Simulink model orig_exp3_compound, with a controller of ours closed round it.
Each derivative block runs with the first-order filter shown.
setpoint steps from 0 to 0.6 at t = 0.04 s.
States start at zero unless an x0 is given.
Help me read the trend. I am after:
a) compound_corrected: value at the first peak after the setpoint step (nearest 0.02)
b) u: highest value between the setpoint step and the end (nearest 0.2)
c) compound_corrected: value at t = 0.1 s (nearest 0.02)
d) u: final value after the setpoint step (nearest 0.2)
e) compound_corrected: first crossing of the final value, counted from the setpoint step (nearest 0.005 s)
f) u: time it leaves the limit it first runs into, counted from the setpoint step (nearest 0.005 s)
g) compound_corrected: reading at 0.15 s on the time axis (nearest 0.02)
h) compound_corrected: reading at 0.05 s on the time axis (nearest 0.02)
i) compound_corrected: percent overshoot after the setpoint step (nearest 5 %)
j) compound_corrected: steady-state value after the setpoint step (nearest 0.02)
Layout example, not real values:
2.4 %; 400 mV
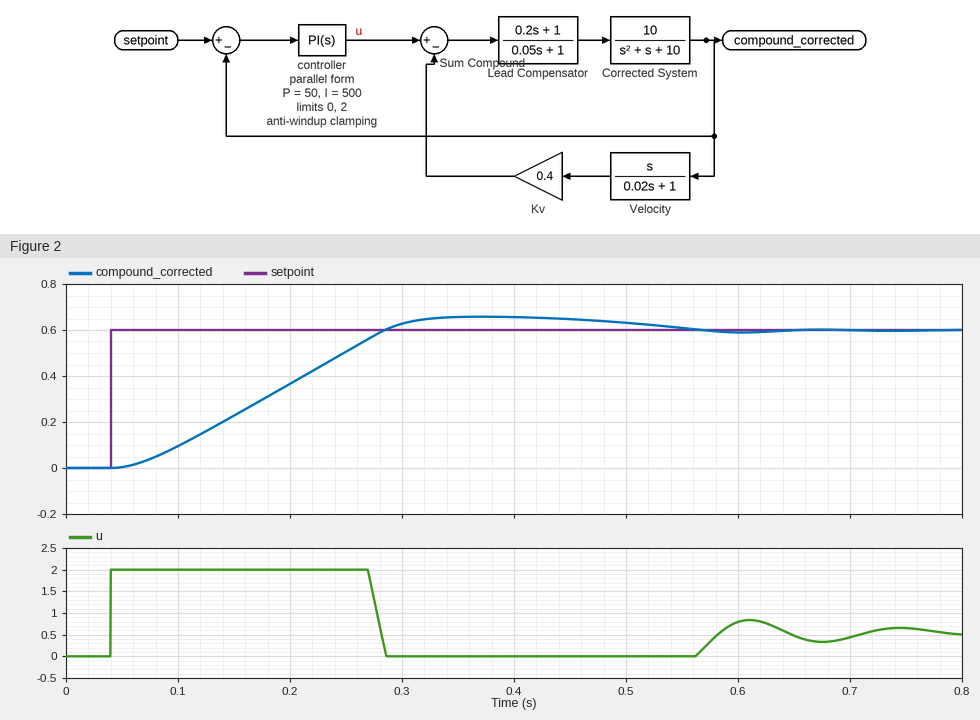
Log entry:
0.66; 2.0; 0.10; 0.6; 0.245 s; 0.230 s; 0.22; 0.00; 10 %; 0.60
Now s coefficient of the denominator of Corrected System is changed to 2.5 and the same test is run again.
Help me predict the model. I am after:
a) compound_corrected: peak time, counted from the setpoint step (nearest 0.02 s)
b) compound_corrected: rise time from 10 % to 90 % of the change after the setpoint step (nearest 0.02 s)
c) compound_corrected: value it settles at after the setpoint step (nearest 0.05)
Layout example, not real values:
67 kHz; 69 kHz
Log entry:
0.32 s; 0.20 s; 0.60
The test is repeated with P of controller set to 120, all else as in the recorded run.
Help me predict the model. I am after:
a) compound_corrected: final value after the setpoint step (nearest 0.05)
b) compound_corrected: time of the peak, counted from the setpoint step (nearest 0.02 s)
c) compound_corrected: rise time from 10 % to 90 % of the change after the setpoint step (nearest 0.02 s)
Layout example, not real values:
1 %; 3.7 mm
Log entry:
0.60; 0.34 s; 0.18 s
